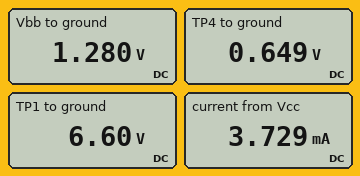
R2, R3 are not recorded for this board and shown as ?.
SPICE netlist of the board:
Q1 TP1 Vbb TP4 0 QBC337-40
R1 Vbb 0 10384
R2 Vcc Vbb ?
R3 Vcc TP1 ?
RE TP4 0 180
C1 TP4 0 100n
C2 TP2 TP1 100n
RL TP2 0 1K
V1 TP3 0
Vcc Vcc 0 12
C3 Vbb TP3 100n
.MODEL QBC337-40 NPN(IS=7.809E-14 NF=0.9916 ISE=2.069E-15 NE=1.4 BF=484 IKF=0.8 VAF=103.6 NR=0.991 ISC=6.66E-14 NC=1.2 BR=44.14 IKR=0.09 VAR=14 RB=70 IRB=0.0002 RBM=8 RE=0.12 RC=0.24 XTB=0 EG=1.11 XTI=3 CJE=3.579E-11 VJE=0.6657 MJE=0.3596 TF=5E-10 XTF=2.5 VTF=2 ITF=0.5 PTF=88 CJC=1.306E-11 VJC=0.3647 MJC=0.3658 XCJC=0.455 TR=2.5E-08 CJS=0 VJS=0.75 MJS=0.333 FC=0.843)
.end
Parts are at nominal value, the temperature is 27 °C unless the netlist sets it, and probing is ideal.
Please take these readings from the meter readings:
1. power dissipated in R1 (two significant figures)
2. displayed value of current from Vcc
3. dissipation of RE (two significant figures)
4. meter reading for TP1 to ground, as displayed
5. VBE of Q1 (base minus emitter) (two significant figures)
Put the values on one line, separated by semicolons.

160 µW; 3.729 mA; 2.3 mW; 6.60 V; 630 mV
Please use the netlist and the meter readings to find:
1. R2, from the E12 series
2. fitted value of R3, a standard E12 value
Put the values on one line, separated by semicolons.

82 kΩ; 1.5 kΩ
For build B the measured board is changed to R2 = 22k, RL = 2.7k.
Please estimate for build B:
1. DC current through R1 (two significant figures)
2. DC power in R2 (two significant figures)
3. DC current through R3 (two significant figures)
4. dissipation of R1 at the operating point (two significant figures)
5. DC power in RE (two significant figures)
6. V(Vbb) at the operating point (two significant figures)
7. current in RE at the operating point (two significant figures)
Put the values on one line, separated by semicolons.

190 µA; 4.5 mW; 7.1 mA; 390 µW; 9.8 mW; 2.0 V; 7.4 mA
